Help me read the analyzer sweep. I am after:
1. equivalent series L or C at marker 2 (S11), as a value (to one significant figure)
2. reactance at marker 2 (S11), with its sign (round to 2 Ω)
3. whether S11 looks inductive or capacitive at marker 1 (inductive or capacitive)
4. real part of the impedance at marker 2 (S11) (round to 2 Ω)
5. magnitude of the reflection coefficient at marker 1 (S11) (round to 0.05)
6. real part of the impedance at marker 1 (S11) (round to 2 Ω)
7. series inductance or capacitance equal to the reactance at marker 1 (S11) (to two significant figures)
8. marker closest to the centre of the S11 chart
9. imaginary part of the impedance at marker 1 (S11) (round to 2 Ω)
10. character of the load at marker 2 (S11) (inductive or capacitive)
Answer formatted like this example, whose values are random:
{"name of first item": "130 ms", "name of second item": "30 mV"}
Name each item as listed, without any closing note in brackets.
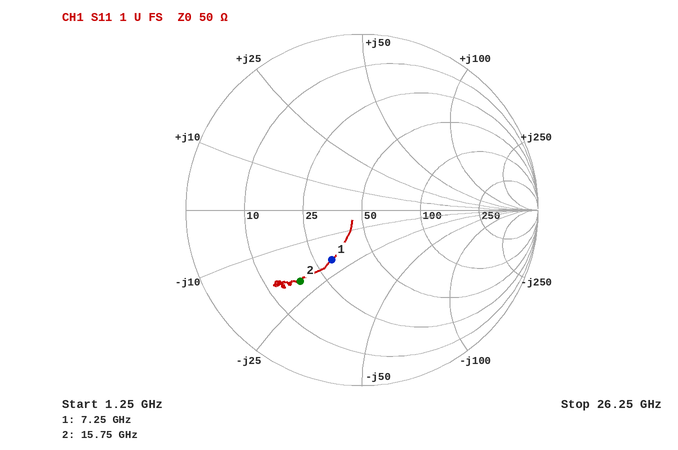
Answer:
{"equivalent series L or C at marker 2 (S11), as a value": "500 fF", "reactance at marker 2 (S11), with its sign": "-20 Ω", "whether S11 looks inductive or capacitive at marker 1": "capacitive", "real part of the impedance at marker 2 (S11)": "18 Ω", "magnitude of the reflection coefficient at marker 1 (S11)": "0.35", "real part of the impedance at marker 1 (S11)": "30 Ω", "series inductance or capacitance equal to the reactance at marker 1 (S11)": "1.1 pF", "marker closest to the centre of the S11 chart": "marker 1", "imaginary part of the impedance at marker 1 (S11)": "-20 Ω", "character of the load at marker 2 (S11)": "capacitive"}
